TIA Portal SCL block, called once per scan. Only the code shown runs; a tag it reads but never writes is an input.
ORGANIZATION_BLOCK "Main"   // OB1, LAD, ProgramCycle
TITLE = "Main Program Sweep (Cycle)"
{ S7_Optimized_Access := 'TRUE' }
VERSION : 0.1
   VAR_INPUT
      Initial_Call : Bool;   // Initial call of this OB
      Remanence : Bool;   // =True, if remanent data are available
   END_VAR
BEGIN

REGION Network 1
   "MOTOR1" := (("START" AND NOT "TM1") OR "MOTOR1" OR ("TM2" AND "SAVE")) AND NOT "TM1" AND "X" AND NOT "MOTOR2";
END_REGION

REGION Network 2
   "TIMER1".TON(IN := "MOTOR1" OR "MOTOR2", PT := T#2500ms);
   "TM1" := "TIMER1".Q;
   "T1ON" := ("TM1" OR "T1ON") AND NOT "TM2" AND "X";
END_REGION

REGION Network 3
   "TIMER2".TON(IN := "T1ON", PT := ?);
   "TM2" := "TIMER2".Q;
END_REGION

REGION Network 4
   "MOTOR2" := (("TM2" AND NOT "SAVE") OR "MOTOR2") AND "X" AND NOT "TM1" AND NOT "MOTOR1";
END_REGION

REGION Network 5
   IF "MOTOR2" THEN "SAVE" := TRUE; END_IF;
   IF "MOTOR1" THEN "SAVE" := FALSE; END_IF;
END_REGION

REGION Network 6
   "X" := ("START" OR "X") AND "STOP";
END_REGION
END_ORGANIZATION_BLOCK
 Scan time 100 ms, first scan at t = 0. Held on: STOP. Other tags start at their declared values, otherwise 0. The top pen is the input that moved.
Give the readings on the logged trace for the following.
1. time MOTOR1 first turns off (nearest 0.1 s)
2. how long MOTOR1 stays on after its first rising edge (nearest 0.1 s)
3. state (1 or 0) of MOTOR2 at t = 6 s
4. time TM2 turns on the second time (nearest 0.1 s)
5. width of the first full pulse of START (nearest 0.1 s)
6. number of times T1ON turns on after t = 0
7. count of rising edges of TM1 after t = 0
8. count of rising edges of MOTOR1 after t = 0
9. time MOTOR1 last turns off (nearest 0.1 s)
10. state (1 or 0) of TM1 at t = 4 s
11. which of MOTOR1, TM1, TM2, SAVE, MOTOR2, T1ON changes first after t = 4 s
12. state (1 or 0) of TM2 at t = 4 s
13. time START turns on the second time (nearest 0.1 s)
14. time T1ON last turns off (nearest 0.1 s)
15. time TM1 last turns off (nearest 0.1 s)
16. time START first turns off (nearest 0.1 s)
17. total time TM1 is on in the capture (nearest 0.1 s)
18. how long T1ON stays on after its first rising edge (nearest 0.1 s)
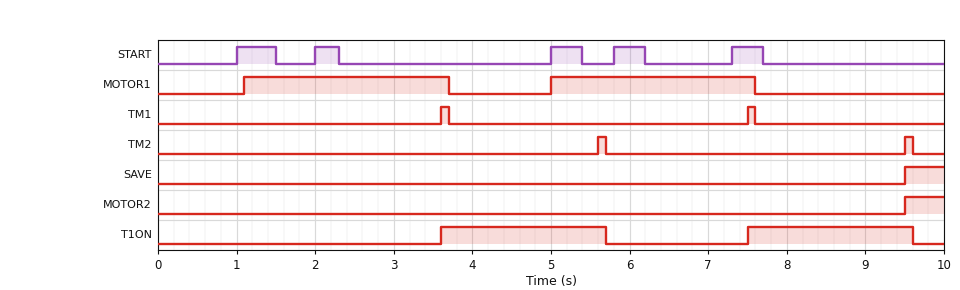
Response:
3.7 s
2.6 s
0
9.5 s
0.5 s
2
2
2
7.6 s
0
MOTOR1
0
2.0 s
9.6 s
7.6 s
1.5 s
0.2 s
2.1 s
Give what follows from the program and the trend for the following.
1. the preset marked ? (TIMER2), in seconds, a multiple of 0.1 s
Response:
2.0 s
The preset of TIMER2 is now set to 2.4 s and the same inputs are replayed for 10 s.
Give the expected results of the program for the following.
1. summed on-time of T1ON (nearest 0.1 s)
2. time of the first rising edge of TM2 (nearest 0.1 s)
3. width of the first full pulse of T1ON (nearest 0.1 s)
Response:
5.0 s
6.0 s
2.5 s
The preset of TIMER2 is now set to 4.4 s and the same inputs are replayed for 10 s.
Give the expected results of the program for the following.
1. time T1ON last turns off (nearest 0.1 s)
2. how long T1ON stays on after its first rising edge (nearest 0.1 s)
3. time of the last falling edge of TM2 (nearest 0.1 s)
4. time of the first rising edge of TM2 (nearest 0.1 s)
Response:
8.1 s
4.5 s
8.1 s
8.0 s
